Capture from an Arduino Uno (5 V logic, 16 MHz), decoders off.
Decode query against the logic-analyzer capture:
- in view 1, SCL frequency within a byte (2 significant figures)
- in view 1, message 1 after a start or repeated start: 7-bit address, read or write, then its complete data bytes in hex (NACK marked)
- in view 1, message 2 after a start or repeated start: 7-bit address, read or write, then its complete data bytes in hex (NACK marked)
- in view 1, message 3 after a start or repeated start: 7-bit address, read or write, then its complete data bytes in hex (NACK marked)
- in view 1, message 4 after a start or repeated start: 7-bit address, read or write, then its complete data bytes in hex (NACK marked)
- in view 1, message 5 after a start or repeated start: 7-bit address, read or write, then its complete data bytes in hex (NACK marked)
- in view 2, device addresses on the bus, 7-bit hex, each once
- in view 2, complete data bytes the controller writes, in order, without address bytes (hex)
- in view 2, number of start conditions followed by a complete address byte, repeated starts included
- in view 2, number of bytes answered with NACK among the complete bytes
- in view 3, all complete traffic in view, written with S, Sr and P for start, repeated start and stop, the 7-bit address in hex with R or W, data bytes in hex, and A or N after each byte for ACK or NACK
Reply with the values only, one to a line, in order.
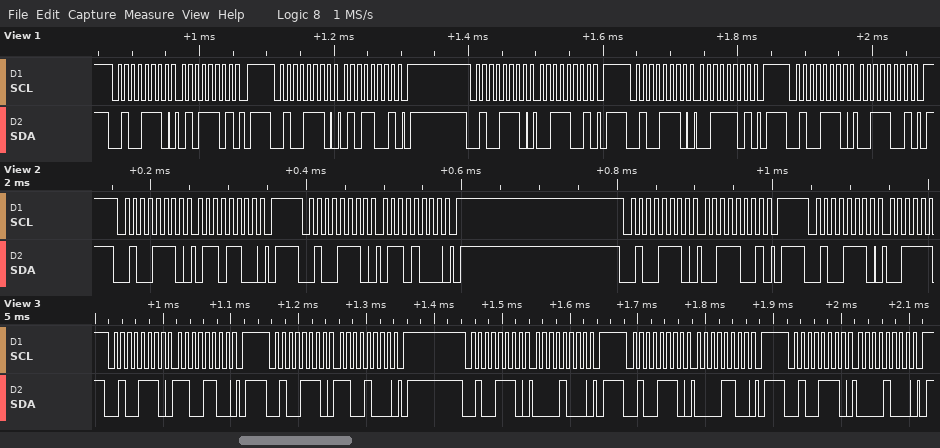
100 kHz
0x27 write: 5D
0x27 write: 59
0x27 write: 39
0x27 write: 3D
0x27 write: 39
0x27
6C 68 39
4
0
S 27W A CC A P S 27W A C8 A P S 27W A 08 A P S 27W A 0C A P S 27W A 08 A P
